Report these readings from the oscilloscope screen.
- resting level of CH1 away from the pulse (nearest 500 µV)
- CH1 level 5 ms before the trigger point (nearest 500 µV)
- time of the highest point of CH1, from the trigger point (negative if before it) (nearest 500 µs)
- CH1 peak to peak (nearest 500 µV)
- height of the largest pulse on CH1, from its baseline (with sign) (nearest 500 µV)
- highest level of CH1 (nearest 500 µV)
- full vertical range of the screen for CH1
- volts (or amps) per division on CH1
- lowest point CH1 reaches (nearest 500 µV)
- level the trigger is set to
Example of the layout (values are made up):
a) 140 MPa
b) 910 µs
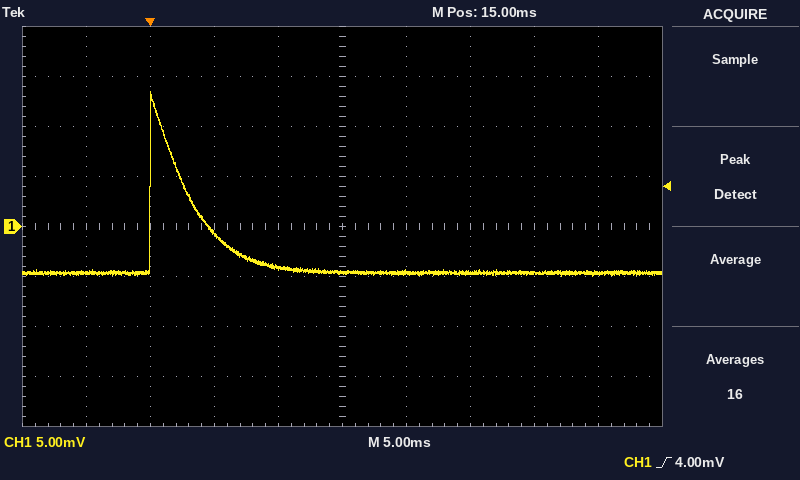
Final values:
a) -4.5 mV
b) -4.5 mV
c) 0.0 ms
d) 18.5 mV
e) +18.0 mV
f) 13.5 mV
g) 40 mV
h) 5 mV
i) -5.0 mV
j) 4.00 mV
